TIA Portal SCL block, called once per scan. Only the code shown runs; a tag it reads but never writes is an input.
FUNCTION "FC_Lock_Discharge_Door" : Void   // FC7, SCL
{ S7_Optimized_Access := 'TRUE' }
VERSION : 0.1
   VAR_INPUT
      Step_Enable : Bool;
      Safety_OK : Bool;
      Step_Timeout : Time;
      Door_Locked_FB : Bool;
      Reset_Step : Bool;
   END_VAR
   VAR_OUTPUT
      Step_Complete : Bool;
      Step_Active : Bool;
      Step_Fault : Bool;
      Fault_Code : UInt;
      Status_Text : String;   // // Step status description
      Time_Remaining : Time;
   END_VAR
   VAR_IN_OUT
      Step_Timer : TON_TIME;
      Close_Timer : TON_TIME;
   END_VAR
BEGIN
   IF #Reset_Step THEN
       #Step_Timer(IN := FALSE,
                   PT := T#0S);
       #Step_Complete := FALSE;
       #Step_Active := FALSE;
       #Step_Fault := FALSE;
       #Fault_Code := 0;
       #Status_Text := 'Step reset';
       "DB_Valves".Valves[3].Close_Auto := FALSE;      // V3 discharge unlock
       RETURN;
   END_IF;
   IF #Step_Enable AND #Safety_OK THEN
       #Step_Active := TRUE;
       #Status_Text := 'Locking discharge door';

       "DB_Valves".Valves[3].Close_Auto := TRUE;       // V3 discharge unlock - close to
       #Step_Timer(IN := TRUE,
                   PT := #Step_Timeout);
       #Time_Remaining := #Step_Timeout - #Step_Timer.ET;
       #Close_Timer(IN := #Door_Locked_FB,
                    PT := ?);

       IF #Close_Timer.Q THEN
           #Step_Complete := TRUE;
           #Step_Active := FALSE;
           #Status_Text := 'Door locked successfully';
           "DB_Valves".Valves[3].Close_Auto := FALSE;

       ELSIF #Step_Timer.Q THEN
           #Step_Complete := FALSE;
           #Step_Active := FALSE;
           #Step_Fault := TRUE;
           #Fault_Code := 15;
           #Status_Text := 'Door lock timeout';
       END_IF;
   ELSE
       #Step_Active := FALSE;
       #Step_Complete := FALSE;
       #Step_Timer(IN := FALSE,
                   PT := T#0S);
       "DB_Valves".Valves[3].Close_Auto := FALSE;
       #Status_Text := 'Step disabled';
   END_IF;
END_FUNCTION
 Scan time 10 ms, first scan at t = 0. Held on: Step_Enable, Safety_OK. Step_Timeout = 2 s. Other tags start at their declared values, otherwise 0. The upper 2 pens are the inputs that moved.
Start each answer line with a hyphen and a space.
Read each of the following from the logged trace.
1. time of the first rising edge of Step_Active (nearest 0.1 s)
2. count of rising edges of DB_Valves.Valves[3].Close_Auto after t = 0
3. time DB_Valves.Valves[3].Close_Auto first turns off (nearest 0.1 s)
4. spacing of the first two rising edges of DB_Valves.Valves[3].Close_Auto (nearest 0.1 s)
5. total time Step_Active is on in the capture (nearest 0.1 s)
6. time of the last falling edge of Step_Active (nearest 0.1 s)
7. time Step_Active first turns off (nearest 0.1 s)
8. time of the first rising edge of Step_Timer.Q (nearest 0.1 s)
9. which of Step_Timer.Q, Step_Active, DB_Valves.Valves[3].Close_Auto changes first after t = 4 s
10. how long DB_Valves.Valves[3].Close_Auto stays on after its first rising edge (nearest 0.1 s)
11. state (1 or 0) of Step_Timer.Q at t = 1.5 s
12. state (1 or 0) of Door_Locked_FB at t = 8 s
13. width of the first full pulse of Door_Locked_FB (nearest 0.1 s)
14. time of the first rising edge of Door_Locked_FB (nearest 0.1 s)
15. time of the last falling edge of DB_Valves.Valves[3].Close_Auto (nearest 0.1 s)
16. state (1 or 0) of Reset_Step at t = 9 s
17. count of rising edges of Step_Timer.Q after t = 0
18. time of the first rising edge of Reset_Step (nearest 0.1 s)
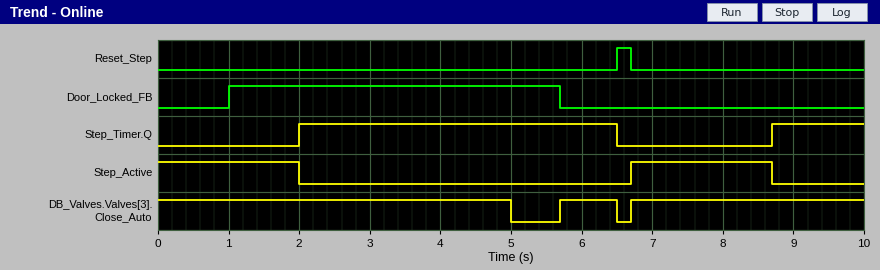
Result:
- 6.7 s
- 2
- 5.0 s
- 1.0 s
- 4.0 s
- 8.7 s
- 2.0 s
- 2.0 s
- DB_Valves.Valves[3].Close_Auto
- 0.8 s
- 0
- 0
- 4.7 s
- 1.0 s
- 6.5 s
- 0
- 2
- 6.5 s
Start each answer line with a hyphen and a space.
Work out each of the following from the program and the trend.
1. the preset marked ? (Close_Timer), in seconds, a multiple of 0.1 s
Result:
- 4.0 s
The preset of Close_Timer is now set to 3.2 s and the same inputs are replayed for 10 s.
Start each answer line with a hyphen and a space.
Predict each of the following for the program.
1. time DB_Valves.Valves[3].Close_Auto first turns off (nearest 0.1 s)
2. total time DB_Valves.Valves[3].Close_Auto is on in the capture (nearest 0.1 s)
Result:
- 4.2 s
- 8.3 s
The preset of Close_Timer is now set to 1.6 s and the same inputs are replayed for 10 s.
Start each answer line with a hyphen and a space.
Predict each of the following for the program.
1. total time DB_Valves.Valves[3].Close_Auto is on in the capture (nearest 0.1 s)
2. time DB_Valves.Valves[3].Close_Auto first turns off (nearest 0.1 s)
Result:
- 6.7 s
- 2.6 s
